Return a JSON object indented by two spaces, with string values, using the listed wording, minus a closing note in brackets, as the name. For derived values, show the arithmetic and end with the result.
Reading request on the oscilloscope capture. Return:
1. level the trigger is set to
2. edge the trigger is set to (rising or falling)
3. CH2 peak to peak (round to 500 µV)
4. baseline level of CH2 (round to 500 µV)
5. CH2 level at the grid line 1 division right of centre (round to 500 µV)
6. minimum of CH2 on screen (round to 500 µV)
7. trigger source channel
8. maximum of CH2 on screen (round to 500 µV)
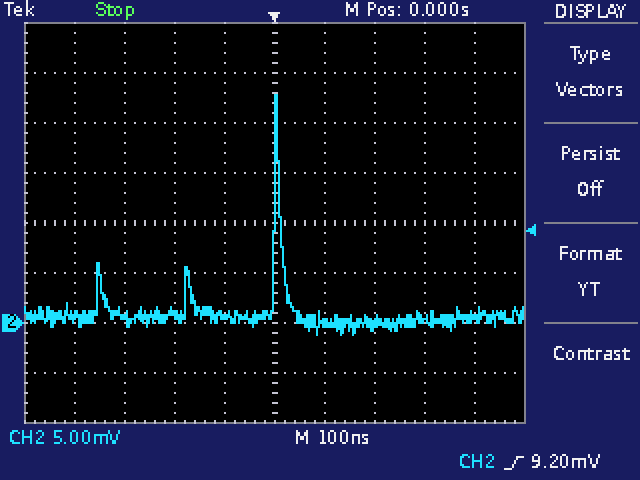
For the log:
{
  "level the trigger is set to": "9.20 mV",
  "edge the trigger is set to": "rising",
  "CH2 peak to peak": "23.0 mV − (-1.0 mV) = 24.0 mV",
  "baseline level of CH2": "500 µV",
  "CH2 level at the grid line 1 division right of centre": "0.0 mV",
  "minimum of CH2 on screen": "-1.0 mV",
  "trigger source channel": "CH2",
  "maximum of CH2 on screen": "23.0 mV"
}
